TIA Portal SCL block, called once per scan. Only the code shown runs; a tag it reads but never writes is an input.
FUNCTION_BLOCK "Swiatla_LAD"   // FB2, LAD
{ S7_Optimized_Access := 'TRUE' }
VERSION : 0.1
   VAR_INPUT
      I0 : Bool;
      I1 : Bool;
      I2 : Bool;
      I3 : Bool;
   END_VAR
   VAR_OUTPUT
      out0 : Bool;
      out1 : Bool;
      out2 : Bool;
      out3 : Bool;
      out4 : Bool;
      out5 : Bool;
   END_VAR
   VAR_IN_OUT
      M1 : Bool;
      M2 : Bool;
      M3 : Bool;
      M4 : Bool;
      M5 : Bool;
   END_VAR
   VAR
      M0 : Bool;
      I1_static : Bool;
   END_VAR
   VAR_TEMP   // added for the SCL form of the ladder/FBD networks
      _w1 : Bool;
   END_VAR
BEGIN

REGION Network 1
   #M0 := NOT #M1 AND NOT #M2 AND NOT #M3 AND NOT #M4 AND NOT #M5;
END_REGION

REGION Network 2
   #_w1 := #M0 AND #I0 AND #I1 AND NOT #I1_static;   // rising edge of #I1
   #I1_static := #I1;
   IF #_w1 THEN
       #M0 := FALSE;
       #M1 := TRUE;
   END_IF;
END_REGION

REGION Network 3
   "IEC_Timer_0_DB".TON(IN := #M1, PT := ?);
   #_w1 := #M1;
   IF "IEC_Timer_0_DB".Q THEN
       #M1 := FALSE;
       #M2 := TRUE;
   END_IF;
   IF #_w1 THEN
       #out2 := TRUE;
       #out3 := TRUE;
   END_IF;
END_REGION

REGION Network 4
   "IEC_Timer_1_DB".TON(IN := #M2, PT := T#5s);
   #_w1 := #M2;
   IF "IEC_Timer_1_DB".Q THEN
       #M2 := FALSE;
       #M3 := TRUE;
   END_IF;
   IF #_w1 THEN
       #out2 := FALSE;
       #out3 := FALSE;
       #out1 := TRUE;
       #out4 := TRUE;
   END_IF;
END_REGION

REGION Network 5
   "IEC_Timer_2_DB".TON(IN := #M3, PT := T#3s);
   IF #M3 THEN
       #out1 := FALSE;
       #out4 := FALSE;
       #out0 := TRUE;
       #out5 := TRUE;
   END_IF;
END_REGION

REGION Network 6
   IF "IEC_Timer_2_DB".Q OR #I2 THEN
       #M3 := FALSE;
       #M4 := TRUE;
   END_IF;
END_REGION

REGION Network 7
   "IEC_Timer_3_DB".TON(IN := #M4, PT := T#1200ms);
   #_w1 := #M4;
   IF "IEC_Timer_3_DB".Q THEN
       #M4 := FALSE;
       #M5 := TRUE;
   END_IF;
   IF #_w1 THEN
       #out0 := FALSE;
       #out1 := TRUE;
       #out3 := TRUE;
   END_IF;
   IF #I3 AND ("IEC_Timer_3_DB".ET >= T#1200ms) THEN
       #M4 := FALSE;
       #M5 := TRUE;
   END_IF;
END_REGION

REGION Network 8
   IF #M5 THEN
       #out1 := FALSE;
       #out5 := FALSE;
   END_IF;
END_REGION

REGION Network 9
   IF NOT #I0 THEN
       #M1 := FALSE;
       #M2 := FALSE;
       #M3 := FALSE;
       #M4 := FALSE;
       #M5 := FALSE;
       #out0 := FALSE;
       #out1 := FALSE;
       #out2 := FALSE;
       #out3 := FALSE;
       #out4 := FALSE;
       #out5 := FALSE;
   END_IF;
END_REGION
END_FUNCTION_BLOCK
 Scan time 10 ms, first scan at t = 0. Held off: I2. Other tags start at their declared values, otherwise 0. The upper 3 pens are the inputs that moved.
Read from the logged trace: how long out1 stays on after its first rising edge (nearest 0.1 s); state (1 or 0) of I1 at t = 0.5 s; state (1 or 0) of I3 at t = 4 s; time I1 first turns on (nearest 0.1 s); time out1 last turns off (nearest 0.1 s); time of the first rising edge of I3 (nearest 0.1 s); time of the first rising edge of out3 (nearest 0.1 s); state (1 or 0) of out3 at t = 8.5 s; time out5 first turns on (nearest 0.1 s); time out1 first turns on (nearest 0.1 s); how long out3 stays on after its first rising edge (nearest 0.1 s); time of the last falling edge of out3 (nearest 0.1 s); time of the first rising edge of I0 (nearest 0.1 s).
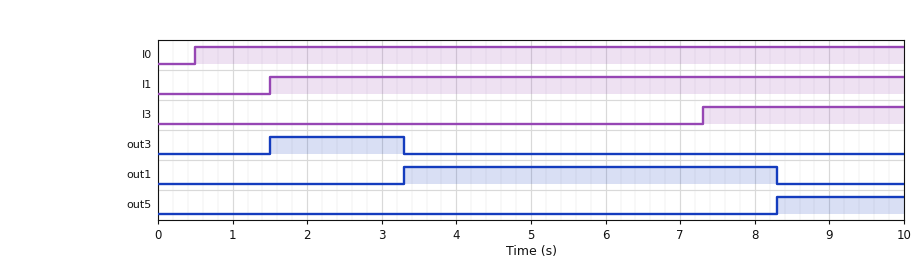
5.0 s
0
0
1.5 s
8.3 s
7.3 s
1.5 s
0
8.3 s
3.3 s
1.8 s
3.3 s
0.5 s
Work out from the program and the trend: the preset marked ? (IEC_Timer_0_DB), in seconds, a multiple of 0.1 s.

1.8 s
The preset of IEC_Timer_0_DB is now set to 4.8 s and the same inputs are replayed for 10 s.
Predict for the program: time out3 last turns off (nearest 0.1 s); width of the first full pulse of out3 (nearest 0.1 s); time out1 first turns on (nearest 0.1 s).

6.3 s
4.8 s
6.3 s
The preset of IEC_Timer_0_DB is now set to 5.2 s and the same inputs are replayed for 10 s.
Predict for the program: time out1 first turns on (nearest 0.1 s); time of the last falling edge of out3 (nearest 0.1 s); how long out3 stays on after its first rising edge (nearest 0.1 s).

6.7 s
6.7 s
5.2 s
